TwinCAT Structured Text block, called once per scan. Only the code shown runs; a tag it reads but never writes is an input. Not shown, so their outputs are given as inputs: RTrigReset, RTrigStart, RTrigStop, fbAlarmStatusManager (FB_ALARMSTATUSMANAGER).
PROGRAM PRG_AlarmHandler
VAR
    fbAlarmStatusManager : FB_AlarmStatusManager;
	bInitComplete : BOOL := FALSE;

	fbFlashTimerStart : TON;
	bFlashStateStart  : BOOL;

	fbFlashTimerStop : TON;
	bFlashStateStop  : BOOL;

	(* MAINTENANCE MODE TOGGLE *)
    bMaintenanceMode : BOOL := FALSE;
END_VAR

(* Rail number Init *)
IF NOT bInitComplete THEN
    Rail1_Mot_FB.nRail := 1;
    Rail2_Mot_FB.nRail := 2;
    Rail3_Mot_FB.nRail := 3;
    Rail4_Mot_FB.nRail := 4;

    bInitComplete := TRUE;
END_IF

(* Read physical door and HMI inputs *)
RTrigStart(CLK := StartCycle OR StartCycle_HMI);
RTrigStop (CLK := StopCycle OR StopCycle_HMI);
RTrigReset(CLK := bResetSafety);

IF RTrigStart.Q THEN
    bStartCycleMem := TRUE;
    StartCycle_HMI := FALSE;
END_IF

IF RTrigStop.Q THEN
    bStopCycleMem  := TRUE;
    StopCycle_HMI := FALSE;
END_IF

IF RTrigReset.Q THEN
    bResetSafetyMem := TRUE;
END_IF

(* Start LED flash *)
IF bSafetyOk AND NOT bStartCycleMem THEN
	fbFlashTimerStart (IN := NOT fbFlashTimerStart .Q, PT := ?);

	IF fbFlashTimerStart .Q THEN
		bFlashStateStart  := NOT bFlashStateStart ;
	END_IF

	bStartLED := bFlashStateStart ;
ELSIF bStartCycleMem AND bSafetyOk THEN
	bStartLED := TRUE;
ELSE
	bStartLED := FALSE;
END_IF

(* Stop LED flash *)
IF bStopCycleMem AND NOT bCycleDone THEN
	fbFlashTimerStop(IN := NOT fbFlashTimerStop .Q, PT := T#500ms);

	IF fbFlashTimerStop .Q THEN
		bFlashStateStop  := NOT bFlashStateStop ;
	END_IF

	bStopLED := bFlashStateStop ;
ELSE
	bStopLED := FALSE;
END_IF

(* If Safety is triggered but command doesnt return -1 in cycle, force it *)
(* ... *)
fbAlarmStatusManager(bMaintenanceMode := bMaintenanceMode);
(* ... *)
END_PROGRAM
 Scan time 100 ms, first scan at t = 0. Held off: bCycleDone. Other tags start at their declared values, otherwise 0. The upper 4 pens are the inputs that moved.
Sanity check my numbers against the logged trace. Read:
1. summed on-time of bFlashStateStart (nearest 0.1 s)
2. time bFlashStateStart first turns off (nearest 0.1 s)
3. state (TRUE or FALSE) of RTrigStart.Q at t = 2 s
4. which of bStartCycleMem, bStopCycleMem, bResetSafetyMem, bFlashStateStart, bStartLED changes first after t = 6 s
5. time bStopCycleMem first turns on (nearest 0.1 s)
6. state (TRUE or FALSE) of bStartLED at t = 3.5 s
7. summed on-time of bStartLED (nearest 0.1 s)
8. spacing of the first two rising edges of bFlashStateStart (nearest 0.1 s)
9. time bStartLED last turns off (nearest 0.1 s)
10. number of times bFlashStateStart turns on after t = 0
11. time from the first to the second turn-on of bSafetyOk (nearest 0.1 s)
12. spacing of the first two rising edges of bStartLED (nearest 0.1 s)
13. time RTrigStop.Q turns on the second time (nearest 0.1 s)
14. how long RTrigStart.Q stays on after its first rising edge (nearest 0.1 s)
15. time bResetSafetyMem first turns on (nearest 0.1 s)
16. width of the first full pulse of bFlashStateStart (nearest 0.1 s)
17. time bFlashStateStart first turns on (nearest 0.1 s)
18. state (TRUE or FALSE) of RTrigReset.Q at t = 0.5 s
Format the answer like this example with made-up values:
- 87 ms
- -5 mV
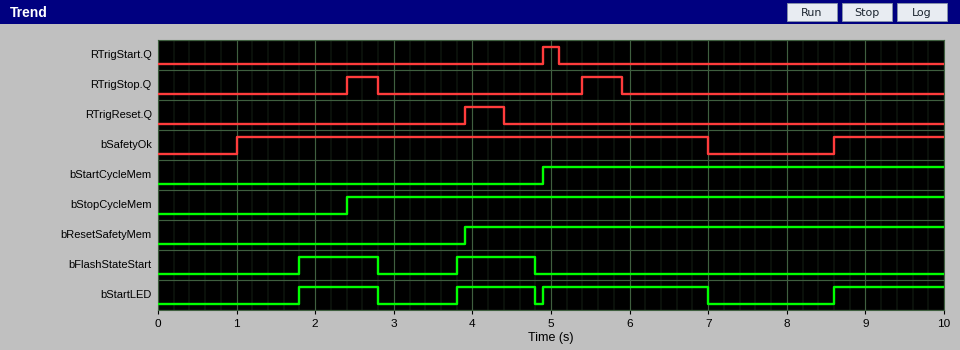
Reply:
- 2.0 s
- 2.8 s
- FALSE
- bStartLED
- 2.4 s
- FALSE
- 5.5 s
- 2.0 s
- 7.0 s
- 2
- 7.6 s
- 2.0 s
- 5.4 s
- 0.2 s
- 3.9 s
- 1.0 s
- 1.8 s
- FALSE
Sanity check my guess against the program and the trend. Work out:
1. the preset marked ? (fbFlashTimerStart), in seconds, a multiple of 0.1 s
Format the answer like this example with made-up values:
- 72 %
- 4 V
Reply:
- 0.8 s
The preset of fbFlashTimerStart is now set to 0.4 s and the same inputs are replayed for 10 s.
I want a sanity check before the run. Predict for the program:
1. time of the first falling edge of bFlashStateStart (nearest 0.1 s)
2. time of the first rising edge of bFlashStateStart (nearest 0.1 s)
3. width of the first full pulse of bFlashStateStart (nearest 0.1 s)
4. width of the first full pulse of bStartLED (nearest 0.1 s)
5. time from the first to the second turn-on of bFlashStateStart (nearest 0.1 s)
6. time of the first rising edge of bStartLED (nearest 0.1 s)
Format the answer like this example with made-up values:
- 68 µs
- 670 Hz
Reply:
- 2.0 s
- 1.4 s
- 0.6 s
- 0.6 s
- 1.2 s
- 1.4 s
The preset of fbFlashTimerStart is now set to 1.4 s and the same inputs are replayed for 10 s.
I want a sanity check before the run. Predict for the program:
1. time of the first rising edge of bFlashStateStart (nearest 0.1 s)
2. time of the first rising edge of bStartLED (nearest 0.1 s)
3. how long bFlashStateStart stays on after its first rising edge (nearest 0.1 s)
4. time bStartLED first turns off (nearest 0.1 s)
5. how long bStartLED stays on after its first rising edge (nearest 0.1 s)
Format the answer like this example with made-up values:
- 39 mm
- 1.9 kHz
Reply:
- 2.4 s
- 2.4 s
- 1.6 s
- 4.0 s
- 1.6 s
